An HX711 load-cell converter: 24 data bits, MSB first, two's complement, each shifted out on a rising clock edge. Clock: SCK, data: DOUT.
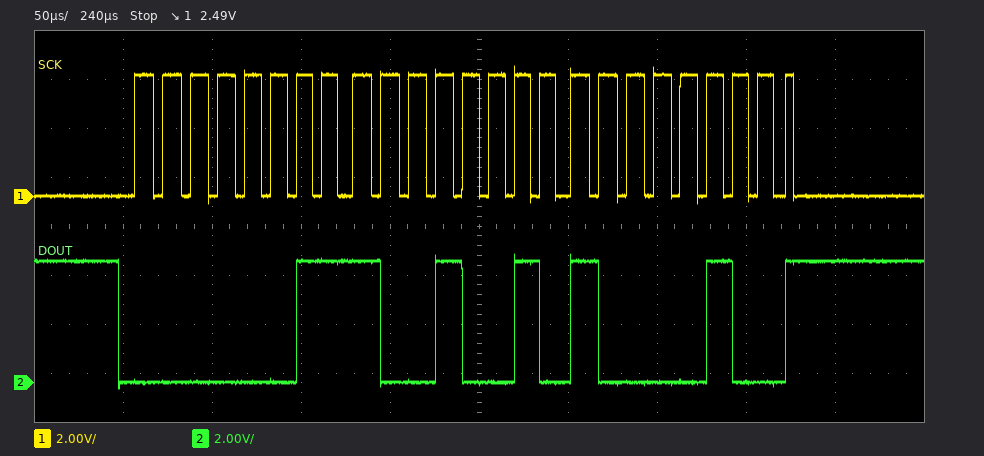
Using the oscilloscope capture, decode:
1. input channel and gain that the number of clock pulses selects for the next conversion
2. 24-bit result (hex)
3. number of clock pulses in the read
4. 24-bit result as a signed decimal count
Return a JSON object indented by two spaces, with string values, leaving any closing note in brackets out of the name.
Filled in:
{
  "input channel and gain that the number of clock pulses selects for the next conversion": "channel A, gain 128",
  "24-bit result": "0x039284",
  "number of clock pulses in the read": "25",
  "24-bit result as a signed decimal count": "234116"
}
